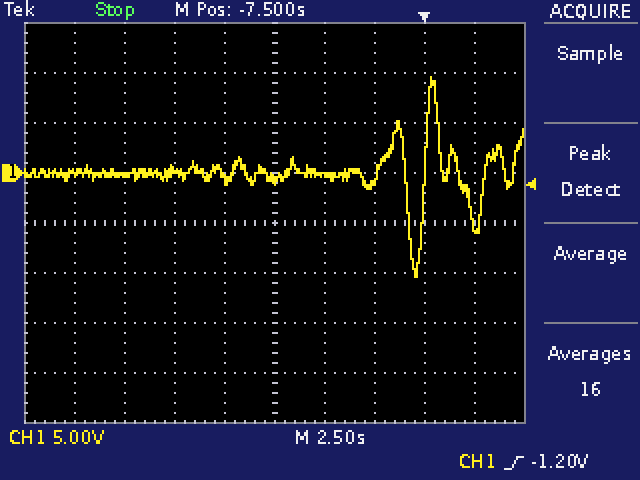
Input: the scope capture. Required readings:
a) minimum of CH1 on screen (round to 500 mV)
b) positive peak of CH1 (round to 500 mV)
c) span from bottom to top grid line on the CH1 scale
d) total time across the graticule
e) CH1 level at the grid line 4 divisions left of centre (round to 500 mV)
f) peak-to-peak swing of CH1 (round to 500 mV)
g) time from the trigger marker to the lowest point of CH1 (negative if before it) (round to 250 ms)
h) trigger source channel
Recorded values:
-10.5 V
9.5 V
40 V
25 s
0.0 V
20.0 V
-500 ms
CH1
